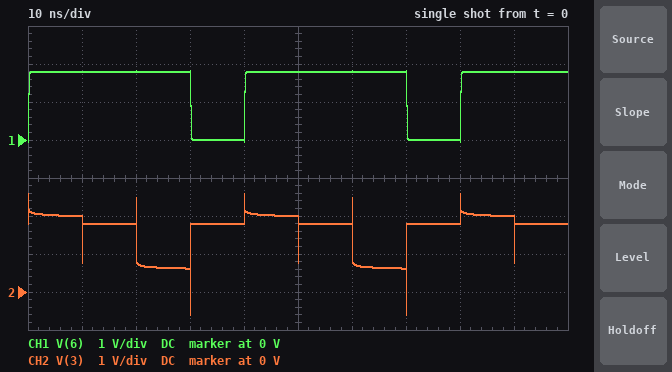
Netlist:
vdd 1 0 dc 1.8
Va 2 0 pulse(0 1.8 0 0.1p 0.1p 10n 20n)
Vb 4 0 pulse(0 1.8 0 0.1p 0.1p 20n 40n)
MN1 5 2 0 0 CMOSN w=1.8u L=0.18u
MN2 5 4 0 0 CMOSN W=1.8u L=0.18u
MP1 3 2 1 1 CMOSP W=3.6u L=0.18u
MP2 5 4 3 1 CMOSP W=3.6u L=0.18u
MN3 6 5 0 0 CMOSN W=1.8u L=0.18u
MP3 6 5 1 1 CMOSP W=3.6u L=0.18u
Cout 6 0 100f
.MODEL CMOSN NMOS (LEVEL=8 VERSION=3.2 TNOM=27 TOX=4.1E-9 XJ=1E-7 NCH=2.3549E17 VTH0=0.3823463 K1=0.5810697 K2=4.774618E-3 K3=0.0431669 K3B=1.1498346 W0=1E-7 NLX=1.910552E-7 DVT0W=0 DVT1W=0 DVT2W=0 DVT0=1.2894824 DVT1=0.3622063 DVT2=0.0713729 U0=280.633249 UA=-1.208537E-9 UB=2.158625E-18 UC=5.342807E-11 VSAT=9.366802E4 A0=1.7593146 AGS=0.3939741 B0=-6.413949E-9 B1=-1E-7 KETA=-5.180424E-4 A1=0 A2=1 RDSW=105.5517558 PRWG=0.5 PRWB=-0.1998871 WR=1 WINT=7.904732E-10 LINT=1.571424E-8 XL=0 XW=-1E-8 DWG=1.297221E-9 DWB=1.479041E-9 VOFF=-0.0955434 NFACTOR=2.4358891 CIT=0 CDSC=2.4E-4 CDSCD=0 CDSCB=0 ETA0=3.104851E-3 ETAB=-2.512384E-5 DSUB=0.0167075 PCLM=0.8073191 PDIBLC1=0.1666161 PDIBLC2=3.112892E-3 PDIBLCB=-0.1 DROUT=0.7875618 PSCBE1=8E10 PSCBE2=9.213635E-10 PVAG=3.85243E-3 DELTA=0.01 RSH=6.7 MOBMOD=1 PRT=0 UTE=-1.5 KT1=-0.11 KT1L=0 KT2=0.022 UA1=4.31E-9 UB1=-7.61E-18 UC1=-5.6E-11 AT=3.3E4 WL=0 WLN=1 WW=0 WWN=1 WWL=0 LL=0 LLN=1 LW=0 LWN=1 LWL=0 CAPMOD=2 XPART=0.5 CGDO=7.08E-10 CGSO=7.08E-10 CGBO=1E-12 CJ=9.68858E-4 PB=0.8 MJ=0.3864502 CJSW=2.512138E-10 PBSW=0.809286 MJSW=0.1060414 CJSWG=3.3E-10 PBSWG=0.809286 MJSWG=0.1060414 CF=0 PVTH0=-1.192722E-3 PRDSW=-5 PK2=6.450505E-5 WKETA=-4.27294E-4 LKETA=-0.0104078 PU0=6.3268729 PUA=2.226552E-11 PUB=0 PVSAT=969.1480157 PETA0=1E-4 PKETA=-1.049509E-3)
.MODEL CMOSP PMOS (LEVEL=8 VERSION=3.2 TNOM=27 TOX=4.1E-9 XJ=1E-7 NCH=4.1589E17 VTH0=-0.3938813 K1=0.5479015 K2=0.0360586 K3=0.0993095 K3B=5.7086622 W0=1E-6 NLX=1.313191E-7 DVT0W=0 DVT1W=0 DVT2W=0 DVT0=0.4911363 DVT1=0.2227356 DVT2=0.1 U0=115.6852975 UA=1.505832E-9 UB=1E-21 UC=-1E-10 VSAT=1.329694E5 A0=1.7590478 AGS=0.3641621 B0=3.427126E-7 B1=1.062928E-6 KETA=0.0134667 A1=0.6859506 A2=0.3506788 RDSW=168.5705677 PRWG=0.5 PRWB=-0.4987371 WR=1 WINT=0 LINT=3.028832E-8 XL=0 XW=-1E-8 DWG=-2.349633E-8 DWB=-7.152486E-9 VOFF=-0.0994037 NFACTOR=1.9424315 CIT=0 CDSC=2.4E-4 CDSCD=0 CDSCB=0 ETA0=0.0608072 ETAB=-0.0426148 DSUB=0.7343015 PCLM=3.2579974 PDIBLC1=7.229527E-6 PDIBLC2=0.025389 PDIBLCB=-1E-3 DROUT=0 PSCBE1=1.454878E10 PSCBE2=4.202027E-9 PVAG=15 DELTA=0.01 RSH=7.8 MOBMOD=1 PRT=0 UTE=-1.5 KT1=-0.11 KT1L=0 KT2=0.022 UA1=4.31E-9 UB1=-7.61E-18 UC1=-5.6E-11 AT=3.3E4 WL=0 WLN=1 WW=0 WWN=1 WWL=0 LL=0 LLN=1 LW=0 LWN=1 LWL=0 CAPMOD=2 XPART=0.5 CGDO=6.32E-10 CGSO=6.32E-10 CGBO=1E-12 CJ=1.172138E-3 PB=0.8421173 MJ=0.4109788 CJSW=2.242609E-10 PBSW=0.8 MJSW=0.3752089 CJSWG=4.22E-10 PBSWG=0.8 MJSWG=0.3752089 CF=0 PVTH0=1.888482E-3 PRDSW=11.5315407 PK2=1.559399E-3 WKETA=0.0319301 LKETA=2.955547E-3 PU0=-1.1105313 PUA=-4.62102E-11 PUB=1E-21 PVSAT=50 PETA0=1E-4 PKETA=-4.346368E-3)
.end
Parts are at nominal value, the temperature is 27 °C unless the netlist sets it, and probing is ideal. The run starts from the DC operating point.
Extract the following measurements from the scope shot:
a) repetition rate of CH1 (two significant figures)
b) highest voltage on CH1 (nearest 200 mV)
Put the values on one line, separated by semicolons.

25 MHz; 1.8 V
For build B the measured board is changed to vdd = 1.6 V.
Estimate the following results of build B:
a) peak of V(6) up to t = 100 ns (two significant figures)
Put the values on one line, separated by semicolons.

1.6 V
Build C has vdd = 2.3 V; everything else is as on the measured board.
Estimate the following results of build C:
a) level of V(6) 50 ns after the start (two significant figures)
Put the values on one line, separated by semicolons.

2.3 V
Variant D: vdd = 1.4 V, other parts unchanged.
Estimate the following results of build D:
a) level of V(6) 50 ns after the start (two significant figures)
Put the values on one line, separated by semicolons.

1.4 V
